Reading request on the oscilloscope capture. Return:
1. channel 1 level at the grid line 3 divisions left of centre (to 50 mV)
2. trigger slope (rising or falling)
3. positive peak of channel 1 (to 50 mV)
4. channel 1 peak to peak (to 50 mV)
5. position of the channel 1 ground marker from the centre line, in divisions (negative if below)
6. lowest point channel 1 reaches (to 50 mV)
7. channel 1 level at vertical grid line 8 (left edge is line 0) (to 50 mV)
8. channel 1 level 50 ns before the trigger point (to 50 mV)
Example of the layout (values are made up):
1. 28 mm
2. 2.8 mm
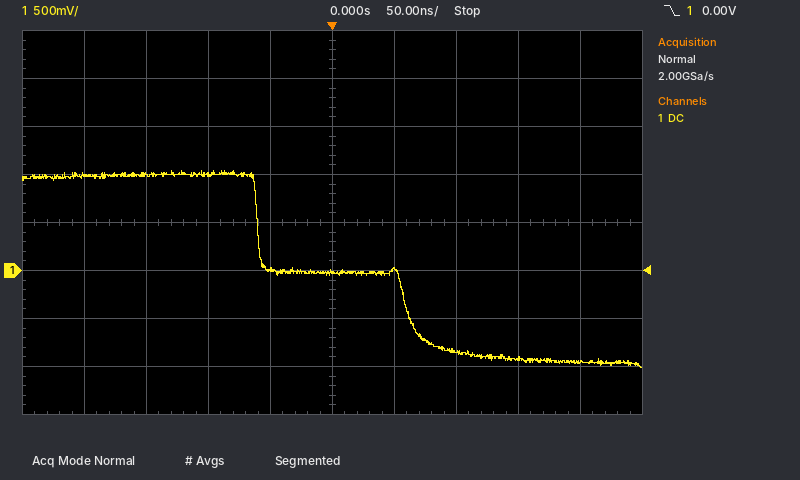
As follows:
1. 1.00 V
2. falling
3. 1.05 V
4. 2.05 V
5. -1.0 div
6. -1.00 V
7. -900 mV
8. 0 mV
